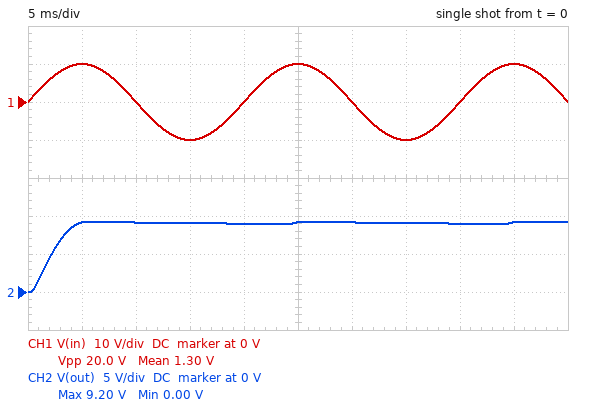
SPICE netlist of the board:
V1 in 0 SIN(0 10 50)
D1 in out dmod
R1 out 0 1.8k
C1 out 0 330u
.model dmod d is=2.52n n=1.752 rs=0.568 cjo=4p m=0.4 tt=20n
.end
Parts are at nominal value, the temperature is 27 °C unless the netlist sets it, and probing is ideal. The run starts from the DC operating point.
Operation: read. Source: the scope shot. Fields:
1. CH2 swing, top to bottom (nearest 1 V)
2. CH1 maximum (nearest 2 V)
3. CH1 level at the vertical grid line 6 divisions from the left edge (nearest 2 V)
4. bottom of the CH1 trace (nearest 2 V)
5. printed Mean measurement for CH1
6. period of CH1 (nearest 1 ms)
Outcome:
9 V
10 V
0 V
-10 V
1.30 V
20 ms
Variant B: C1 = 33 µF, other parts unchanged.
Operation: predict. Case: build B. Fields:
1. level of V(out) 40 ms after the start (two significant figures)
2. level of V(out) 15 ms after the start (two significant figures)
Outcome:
7.3 V
7.9 V
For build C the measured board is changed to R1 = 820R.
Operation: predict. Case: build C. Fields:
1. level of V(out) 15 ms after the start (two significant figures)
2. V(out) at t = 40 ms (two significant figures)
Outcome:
8.9 V
8.7 V
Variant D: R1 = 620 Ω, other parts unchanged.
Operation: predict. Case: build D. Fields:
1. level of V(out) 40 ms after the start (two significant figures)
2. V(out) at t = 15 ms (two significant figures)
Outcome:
8.6 V
8.8 V
